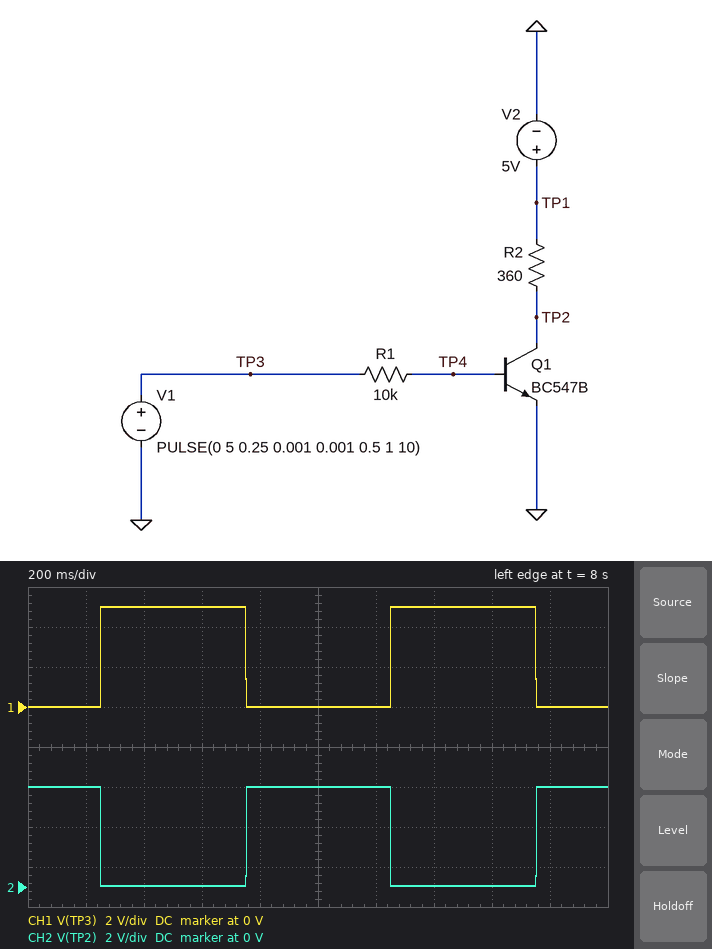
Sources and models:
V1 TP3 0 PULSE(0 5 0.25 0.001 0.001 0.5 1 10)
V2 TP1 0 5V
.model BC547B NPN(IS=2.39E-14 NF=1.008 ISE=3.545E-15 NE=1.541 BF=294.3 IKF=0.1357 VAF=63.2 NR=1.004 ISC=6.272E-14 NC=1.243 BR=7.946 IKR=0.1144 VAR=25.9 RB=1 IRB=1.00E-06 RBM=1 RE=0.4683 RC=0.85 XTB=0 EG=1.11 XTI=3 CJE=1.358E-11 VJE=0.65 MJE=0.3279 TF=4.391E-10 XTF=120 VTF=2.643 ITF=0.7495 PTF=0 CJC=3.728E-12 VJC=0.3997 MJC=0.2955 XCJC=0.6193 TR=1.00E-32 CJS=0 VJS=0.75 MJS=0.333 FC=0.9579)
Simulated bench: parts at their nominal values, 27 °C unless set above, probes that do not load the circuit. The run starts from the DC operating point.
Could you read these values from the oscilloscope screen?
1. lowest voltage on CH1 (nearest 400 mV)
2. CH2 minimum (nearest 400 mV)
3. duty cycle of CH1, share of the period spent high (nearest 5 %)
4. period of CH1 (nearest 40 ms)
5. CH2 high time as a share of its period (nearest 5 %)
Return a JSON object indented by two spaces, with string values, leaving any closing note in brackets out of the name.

{
  "lowest voltage on CH1": "0 V",
  "CH2 minimum": "0 V",
  "duty cycle of CH1, share of the period spent high": "50 %",
  "period of CH1": "1.00 s",
  "CH2 high time as a share of its period": "50 %"
}
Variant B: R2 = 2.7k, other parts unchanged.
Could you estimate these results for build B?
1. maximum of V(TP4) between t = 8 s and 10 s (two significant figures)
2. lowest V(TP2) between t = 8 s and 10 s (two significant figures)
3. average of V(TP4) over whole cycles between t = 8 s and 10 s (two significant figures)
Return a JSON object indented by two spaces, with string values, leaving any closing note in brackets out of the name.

{
  "maximum of V(TP4) between t = 8 s and 10 s": "680 mV",
  "lowest V(TP2) between t = 8 s and 10 s": "22 mV",
  "average of V(TP4) over whole cycles between t = 8 s and 10 s": "340 mV"
}
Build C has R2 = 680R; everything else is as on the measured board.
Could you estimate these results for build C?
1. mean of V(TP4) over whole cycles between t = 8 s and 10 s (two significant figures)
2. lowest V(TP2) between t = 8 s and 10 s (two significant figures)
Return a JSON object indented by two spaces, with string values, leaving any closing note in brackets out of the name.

{
  "mean of V(TP4) over whole cycles between t = 8 s and 10 s": "350 mV",
  "lowest V(TP2) between t = 8 s and 10 s": "50 mV"
}
